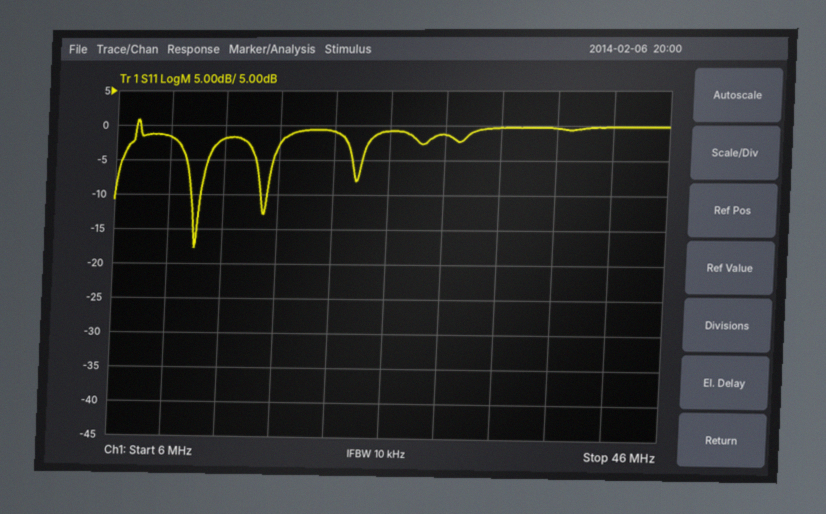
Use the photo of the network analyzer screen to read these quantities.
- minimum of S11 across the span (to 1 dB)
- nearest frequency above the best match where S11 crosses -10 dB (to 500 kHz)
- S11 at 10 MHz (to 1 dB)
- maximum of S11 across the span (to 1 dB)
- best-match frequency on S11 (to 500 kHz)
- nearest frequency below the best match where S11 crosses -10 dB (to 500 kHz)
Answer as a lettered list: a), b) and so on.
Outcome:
a) -18 dB
b) 12.5 MHz
c) -2 dB
d) 1 dB
e) 12.0 MHz
f) 11.5 MHz
